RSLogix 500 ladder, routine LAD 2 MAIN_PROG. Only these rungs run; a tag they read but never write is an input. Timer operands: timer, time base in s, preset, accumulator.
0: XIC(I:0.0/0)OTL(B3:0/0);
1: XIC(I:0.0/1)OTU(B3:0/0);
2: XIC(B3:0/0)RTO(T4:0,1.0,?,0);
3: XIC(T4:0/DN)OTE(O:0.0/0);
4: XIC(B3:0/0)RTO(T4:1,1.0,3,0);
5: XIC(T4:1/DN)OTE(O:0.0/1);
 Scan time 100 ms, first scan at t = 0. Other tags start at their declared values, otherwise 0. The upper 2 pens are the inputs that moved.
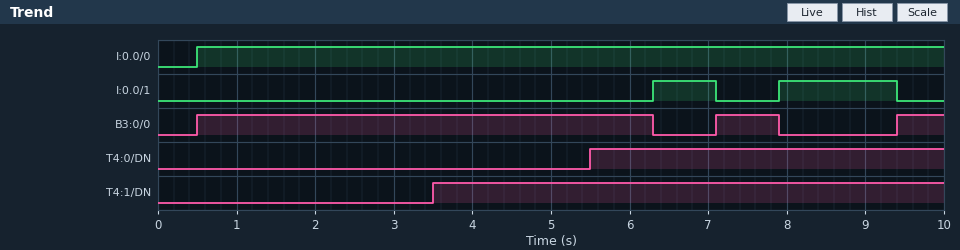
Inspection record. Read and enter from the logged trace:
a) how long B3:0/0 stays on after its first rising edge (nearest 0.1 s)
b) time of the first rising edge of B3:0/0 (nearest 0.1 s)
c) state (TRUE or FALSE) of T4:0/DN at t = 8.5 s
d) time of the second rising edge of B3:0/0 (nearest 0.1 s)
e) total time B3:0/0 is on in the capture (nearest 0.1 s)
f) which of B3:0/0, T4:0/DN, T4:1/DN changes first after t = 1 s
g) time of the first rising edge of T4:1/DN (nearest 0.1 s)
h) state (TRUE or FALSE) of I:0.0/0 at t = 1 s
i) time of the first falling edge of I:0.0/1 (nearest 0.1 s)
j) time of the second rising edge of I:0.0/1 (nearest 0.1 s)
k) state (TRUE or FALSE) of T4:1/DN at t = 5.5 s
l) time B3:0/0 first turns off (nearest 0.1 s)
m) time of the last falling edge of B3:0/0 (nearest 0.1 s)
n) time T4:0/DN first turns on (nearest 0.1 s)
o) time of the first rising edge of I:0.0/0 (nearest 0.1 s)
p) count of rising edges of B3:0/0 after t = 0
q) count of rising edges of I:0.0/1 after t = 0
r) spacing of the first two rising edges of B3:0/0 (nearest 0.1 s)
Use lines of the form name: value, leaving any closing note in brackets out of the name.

how long B3:0/0 stays on after its first rising edge: 5.8 s
time of the first rising edge of B3:0/0: 0.5 s
state (TRUE or FALSE) of T4:0/DN at t = 8.5 s: TRUE
time of the second rising edge of B3:0/0: 7.1 s
total time B3:0/0 is on in the capture: 7.2 s
which of B3:0/0, T4:0/DN, T4:1/DN changes first after t = 1 s: T4:1/DN
time of the first rising edge of T4:1/DN: 3.5 s
state (TRUE or FALSE) of I:0.0/0 at t = 1 s: TRUE
time of the first falling edge of I:0.0/1: 7.1 s
time of the second rising edge of I:0.0/1: 7.9 s
state (TRUE or FALSE) of T4:1/DN at t = 5.5 s: TRUE
time B3:0/0 first turns off: 6.3 s
time of the last falling edge of B3:0/0: 7.9 s
time T4:0/DN first turns on: 5.5 s
time of the first rising edge of I:0.0/0: 0.5 s
count of rising edges of B3:0/0 after t = 0: 3
count of rising edges of I:0.0/1 after t = 0: 2
spacing of the first two rising edges of B3:0/0: 6.6 s
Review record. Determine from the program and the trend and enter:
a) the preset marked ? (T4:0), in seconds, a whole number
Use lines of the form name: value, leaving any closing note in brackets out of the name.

the preset marked ? (T4:0), in seconds, a whole number: 5 s
